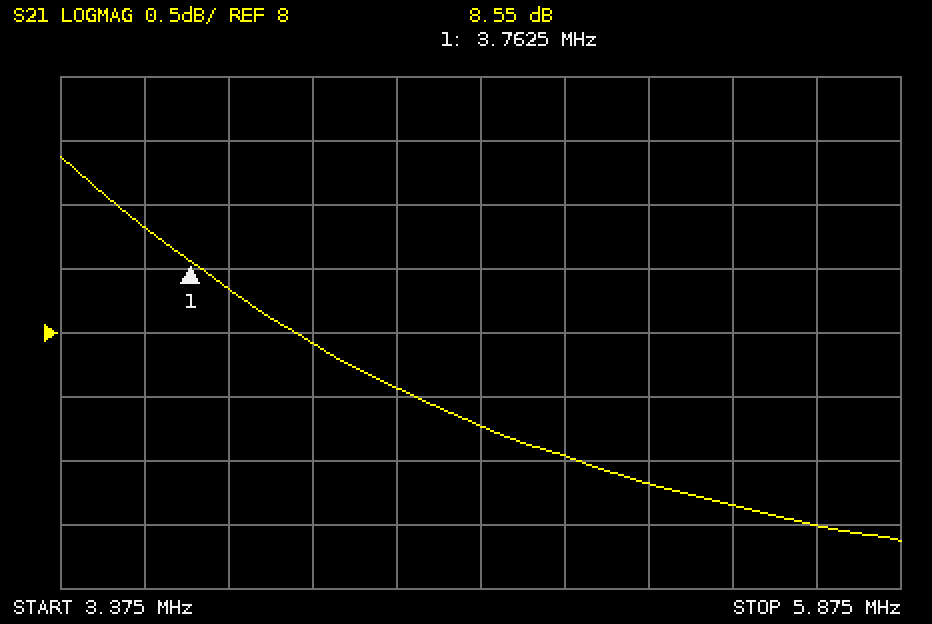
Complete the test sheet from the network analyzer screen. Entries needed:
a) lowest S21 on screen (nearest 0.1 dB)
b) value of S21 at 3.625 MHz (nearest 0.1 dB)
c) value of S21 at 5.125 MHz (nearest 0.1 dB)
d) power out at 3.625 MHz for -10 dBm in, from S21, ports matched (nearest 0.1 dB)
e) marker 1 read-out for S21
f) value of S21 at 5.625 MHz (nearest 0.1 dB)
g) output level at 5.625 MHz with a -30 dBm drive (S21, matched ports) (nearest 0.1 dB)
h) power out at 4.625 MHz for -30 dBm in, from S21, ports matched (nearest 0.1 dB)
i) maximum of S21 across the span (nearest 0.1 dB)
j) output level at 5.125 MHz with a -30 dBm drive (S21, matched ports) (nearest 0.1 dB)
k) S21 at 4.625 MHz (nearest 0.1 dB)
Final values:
6.4 dB
8.8 dB
6.8 dB
-1.2 dBm
8.55 dB
6.5 dB
-23.5 dBm
-22.7 dBm
9.4 dB
-23.2 dBm
7.3 dB
